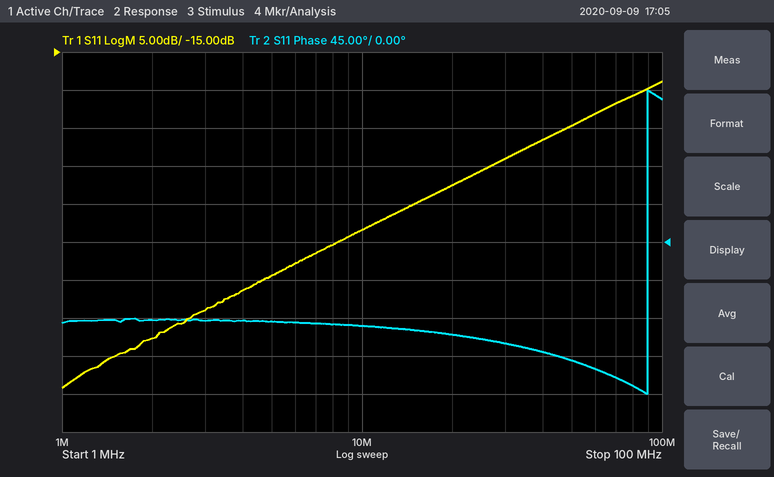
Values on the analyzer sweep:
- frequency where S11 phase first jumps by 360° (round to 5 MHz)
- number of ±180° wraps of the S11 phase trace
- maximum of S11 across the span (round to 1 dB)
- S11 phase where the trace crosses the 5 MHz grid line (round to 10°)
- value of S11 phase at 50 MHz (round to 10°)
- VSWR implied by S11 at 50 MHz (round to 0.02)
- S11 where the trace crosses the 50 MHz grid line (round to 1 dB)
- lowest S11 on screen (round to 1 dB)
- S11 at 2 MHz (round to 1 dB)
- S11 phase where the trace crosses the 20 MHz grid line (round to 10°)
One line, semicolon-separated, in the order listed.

90 MHz; 1; -19 dB; -90°; -140°; 1.12; -25 dB; -59 dB; -53 dB; -110°
